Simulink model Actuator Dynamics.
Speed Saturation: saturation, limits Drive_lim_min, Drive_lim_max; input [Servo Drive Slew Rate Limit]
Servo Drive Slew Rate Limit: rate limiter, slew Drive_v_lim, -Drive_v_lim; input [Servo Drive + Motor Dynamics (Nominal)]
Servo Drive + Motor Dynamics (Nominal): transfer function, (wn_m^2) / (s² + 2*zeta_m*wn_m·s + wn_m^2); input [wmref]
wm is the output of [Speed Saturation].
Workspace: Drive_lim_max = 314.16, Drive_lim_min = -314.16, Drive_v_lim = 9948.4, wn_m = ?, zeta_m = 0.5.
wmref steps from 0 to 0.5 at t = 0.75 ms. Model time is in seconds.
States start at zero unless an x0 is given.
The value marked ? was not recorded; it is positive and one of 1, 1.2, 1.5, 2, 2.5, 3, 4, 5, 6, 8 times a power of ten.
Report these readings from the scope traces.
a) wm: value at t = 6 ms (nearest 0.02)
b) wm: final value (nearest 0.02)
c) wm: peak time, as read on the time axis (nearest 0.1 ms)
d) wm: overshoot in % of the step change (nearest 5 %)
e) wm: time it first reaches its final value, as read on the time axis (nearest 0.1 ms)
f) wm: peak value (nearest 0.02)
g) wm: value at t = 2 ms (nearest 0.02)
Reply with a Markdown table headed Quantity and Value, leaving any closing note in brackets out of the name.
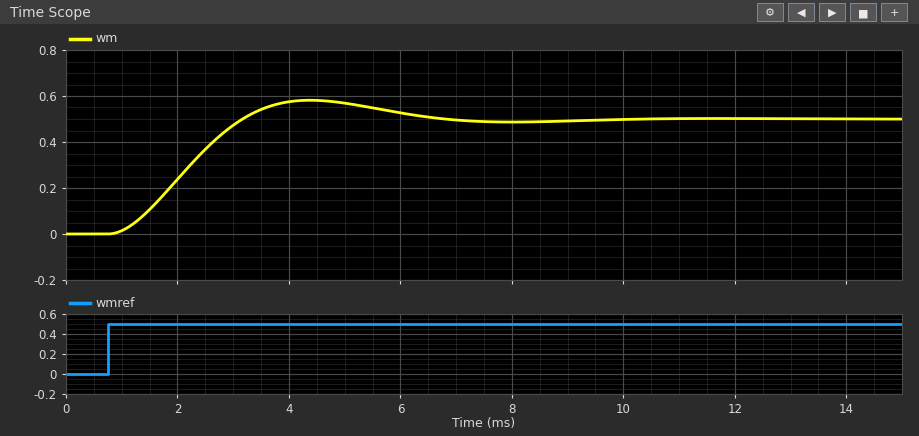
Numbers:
| Quantity | Value |
|---|---|
| wm: value at t = 6 ms | 0.52 |
| wm: final value | 0.50 |
| wm: peak time, as read on the time axis | 4.4 ms |
| wm: overshoot in % of the step change | 15 % |
| wm: time it first reaches its final value, as read on the time axis | 3.2 ms |
| wm: peak value | 0.58 |
| wm: value at t = 2 ms | 0.24 |
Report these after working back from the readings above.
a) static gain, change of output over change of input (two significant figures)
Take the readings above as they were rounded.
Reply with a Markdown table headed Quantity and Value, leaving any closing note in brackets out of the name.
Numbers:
| Quantity | Value |
|---|---|
| static gain, change of output over change of input | 1.0 |
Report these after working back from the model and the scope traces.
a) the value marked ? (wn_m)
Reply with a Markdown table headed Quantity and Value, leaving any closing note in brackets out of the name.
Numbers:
| Quantity | Value |
|---|---|
| the value marked ? | 1000 |
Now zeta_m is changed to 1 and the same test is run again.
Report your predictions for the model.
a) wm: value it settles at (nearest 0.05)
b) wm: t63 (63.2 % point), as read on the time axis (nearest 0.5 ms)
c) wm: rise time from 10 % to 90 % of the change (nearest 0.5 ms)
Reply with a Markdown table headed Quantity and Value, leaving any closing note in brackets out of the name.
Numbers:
| Quantity | Value |
|---|---|
| wm: value it settles at | 0.50 |
| wm: t63 (63.2 % point), as read on the time axis | 3.0 ms |
| wm: rise time from 10 % to 90 % of the change | 3.5 ms |
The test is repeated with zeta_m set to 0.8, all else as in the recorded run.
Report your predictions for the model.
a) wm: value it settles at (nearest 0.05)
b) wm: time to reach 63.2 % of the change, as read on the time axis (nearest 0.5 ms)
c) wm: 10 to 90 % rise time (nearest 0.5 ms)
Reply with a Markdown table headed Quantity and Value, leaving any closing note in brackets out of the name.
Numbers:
| Quantity | Value |
|---|---|
| wm: value it settles at | 0.50 |
| wm: time to reach 63.2 % of the change, as read on the time axis | 2.5 ms |
| wm: 10 to 90 % rise time | 2.5 ms |
